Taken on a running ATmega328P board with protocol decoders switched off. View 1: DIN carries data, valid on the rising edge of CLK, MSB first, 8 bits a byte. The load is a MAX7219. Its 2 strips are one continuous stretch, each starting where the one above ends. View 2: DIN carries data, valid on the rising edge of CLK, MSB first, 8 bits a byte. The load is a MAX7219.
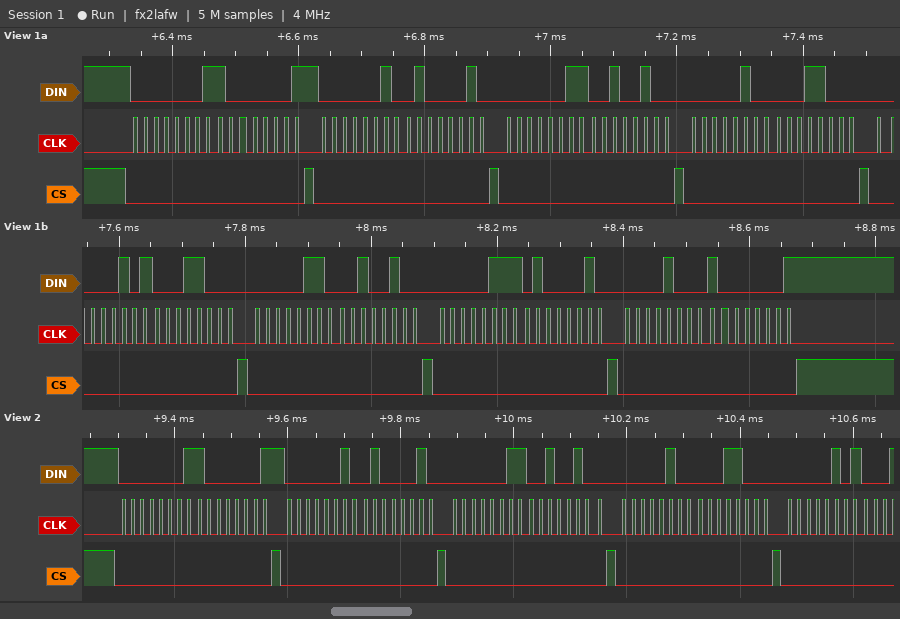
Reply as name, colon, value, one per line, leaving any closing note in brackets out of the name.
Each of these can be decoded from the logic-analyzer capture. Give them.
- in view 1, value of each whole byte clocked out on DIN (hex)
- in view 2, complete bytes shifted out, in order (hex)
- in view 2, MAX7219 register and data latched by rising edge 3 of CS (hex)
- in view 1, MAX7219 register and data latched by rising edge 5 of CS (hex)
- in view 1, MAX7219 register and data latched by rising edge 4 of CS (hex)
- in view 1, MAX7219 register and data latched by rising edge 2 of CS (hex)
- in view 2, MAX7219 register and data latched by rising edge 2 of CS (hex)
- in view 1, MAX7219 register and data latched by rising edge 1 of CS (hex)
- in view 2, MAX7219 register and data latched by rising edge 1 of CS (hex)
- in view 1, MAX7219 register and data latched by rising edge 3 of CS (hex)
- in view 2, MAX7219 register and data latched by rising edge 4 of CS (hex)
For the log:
in view 1, value of each whole byte clocked out on DIN: 01 81 02 42 03 24 04 18 05 18 06 24 07 42 08 81
in view 2, complete bytes shifted out, in order: 0x01 0x81 0x02 0x42 0x03 0x24 0x04 0x18 0x05
in view 2, MAX7219 register and data latched by rising edge 3 of CS: register 0x3, data 0x24
in view 1, MAX7219 register and data latched by rising edge 5 of CS: register 0x5, data 0x18
in view 1, MAX7219 register and data latched by rising edge 4 of CS: register 0x4, data 0x18
in view 1, MAX7219 register and data latched by rising edge 2 of CS: register 0x2, data 0x42
in view 2, MAX7219 register and data latched by rising edge 2 of CS: register 0x2, data 0x42
in view 1, MAX7219 register and data latched by rising edge 1 of CS: register 0x1, data 0x81
in view 2, MAX7219 register and data latched by rising edge 1 of CS: register 0x1, data 0x81
in view 1, MAX7219 register and data latched by rising edge 3 of CS: register 0x3, data 0x24
in view 2, MAX7219 register and data latched by rising edge 4 of CS: register 0x4, data 0x18
